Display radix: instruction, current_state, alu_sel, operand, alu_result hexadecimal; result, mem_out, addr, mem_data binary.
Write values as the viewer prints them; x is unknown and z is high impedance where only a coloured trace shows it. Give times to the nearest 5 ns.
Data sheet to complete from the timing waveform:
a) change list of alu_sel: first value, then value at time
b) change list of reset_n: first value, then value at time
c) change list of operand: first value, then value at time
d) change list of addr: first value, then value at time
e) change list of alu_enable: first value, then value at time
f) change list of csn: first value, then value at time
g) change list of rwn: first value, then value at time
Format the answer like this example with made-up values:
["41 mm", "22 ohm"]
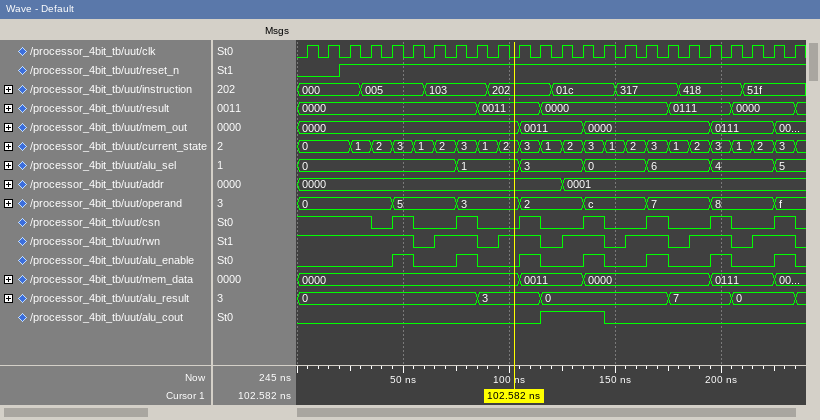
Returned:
["0, 1 at 75 ns, 3 at 105 ns, 0 at 135 ns, 6 at 165 ns, 4 at 195 ns, 5 at 225 ns", "0, 1 at 20 ns", "0, 5 at 45 ns, 3 at 75 ns, 2 at 105 ns, c at 135 ns, 7 at 165 ns, 8 at 195 ns, f at 225 ns", "0000, 0001 at 125 ns", "0, 1 at 45 ns, 0 at 55 ns, 1 at 75 ns, 0 at 85 ns, 1 at 105 ns, 0 at 115 ns, 1 at 135 ns, 0 at 145 ns, 1 at 165 ns, 0 at 175 ns, 1 at 195 ns, 0 at 205 ns, 1 at 225 ns, 0 at 235 ns", "1, 0 at 35 ns, 1 at 45 ns, 0 at 55 ns, 1 at 75 ns, 0 at 85 ns, 1 at 105 ns, 0 at 115 ns, 1 at 135 ns, 0 at 145 ns, 1 at 165 ns, 0 at 175 ns, 1 at 195 ns, 0 at 205 ns, 1 at 225 ns, 0 at 235 ns", "1, 0 at 55 ns, 1 at 65 ns, 0 at 85 ns, 1 at 95 ns, 0 at 115 ns, 1 at 125 ns, 0 at 145 ns, 1 at 155 ns, 0 at 175 ns, 1 at 185 ns, 0 at 205 ns, 1 at 215 ns, 0 at 235 ns"]
